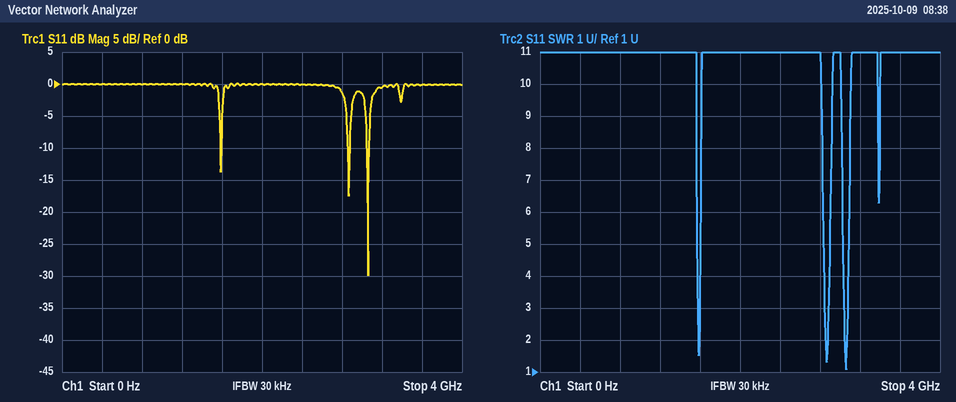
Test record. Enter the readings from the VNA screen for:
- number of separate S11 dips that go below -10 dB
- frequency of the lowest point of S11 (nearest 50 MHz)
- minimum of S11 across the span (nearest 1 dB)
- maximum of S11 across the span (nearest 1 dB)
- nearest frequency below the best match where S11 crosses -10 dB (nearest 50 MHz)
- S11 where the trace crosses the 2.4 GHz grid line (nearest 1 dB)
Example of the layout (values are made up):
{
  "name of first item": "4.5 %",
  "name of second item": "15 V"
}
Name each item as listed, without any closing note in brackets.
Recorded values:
{
  "number of separate S11 dips that go below -10 dB": "3",
  "frequency of the lowest point of S11": "3.05 GHz",
  "minimum of S11 across the span": "-30 dB",
  "maximum of S11 across the span": "0 dB",
  "nearest frequency below the best match where S11 crosses -10 dB": "3.05 GHz",
  "S11 where the trace crosses the 2.4 GHz grid line": "0 dB"
}
